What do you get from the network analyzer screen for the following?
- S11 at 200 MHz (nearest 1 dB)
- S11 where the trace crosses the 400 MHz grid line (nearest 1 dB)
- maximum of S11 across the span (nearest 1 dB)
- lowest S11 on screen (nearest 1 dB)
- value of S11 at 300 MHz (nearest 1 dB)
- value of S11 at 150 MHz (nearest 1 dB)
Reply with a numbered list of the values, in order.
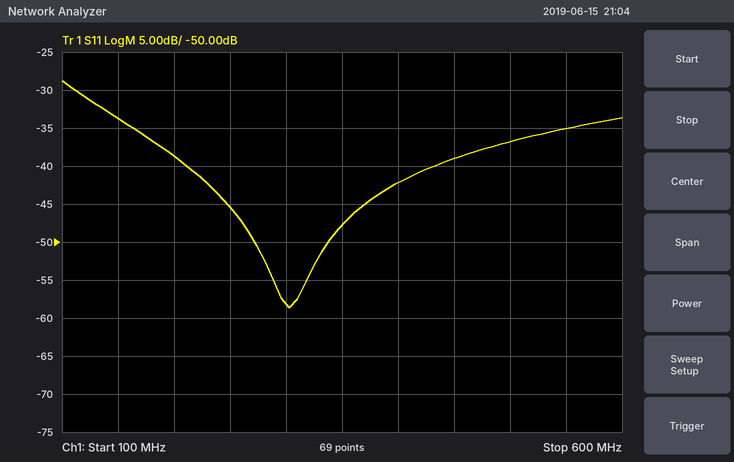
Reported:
1. -39 dB
2. -42 dB
3. -29 dB
4. -59 dB
5. -58 dB
6. -34 dB
